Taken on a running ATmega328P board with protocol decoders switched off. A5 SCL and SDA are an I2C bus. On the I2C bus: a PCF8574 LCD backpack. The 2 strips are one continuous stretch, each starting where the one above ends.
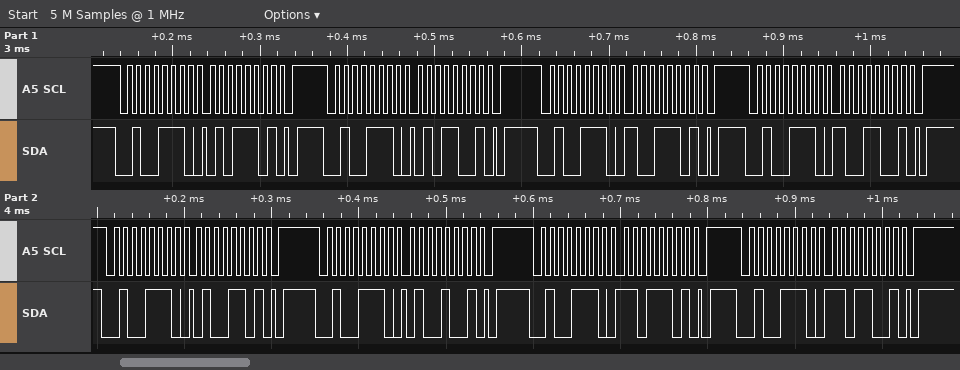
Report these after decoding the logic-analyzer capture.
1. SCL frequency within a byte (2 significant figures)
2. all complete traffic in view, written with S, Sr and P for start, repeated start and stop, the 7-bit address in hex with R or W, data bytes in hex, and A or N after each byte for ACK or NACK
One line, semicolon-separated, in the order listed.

100 kHz; S 27W A 5D A P S 27W A 59 A P S 27W A 9D A P S 27W A 99 A P S 27W A 4D A P S 27W A 49 A P S 27W A DD A P S 27W A D9 A P
